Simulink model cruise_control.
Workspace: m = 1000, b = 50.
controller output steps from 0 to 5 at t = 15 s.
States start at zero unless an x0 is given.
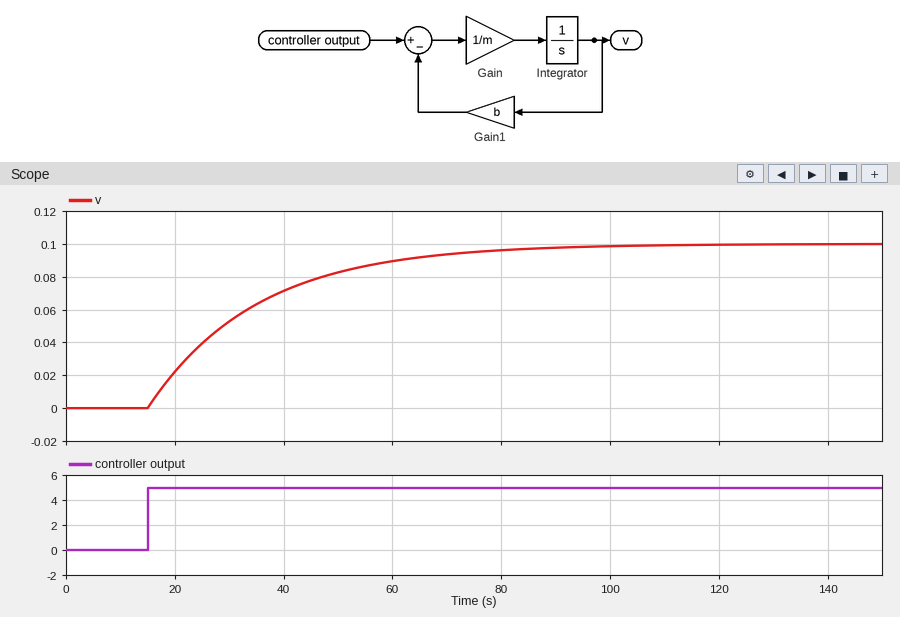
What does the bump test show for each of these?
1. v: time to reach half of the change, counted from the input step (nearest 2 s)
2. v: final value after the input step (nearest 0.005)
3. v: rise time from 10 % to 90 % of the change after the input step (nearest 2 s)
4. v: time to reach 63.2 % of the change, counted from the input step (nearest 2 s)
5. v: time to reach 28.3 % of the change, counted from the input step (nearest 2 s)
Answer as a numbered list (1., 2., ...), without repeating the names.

1. 14 s
2. 0.100
3. 44 s
4. 20 s
5. 6 s
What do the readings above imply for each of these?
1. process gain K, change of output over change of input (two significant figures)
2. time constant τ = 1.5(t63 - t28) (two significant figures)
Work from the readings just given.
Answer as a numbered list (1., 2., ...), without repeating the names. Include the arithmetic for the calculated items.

1. (0.1 - 0) / 5 = 0.020
2. 1.5 × (20 - 6) = 21 s
